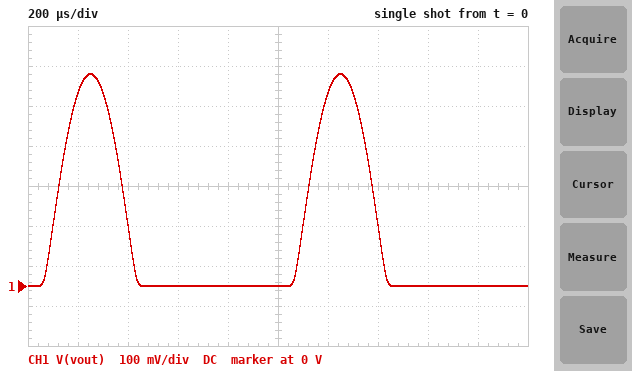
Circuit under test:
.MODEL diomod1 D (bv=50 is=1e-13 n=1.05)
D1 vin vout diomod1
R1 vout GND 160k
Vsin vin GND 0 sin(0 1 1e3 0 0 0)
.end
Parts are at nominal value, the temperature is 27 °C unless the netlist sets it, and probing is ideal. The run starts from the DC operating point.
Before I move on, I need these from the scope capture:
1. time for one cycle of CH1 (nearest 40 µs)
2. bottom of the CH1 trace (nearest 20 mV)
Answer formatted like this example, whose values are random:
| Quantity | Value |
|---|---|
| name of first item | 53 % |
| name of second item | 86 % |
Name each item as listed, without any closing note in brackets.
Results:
| Quantity | Value |
|---|---|
| time for one cycle of CH1 | 1.00 ms |
| bottom of the CH1 trace | 0 V |
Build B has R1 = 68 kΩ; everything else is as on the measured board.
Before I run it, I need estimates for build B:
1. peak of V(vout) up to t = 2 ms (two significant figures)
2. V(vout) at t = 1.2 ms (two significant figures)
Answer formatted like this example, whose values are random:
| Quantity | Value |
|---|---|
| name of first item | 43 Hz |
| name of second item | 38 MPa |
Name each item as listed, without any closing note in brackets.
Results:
| Quantity | Value |
|---|---|
| peak of V(vout) up to t = 2 ms | 510 mV |
| V(vout) at t = 1.2 ms | 460 mV |
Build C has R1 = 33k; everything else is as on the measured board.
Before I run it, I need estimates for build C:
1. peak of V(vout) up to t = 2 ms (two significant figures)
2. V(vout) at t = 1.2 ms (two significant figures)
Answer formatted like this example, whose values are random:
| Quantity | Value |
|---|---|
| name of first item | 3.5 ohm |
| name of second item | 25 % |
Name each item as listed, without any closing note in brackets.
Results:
| Quantity | Value |
|---|---|
| peak of V(vout) up to t = 2 ms | 490 mV |
| V(vout) at t = 1.2 ms | 440 mV |
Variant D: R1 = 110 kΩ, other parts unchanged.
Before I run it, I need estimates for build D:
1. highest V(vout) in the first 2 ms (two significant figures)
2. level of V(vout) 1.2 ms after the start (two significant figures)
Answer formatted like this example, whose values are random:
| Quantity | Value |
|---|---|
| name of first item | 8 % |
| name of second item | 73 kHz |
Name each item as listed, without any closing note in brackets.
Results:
| Quantity | Value |
|---|---|
| highest V(vout) in the first 2 ms | 520 mV |
| level of V(vout) 1.2 ms after the start | 470 mV |
